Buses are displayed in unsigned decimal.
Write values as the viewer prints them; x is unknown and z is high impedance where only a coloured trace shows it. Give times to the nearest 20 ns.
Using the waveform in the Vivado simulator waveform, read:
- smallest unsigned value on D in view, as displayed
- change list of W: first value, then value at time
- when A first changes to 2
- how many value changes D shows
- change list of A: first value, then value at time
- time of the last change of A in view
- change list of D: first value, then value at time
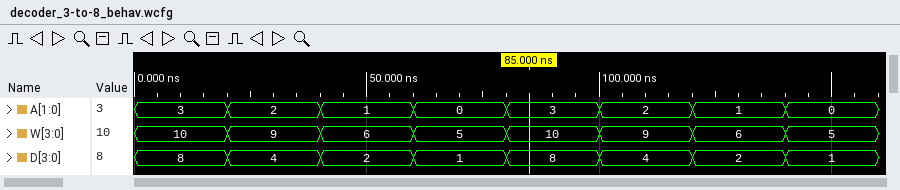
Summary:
1
10, 9 at 20 ns, 6 at 40 ns, 5 at 60 ns, 10 at 80 ns, 9 at 100 ns, 6 at 120 ns, 5 at 140 ns
20 ns
7
3, 2 at 20 ns, 1 at 40 ns, 0 at 60 ns, 3 at 80 ns, 2 at 100 ns, 1 at 120 ns, 0 at 140 ns
140 ns
8, 4 at 20 ns, 2 at 40 ns, 1 at 60 ns, 8 at 80 ns, 4 at 100 ns, 2 at 120 ns, 1 at 140 ns
